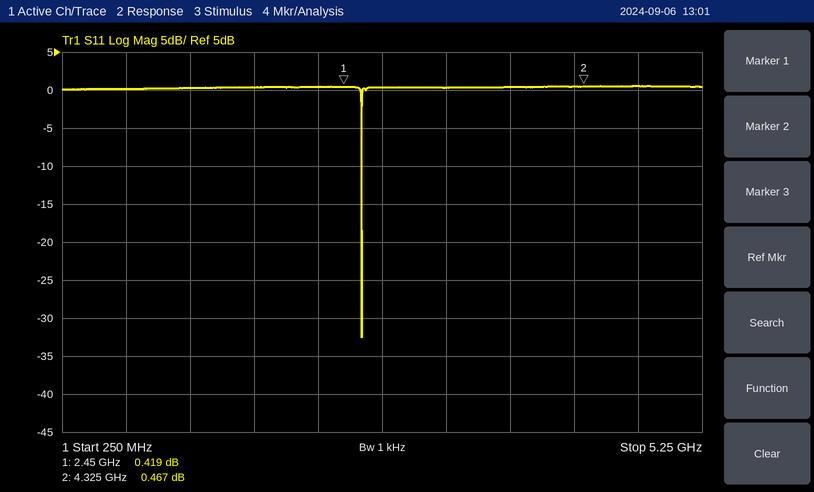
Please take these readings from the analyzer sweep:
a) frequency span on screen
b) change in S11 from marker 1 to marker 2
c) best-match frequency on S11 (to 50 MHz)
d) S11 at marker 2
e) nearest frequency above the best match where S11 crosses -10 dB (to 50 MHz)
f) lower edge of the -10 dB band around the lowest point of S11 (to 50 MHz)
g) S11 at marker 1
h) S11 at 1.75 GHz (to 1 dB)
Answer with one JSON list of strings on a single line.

["5 GHz", "0.048 dB", "2.60 GHz", "0.467 dB", "2.60 GHz", "2.60 GHz", "0.419 dB", "0 dB"]
